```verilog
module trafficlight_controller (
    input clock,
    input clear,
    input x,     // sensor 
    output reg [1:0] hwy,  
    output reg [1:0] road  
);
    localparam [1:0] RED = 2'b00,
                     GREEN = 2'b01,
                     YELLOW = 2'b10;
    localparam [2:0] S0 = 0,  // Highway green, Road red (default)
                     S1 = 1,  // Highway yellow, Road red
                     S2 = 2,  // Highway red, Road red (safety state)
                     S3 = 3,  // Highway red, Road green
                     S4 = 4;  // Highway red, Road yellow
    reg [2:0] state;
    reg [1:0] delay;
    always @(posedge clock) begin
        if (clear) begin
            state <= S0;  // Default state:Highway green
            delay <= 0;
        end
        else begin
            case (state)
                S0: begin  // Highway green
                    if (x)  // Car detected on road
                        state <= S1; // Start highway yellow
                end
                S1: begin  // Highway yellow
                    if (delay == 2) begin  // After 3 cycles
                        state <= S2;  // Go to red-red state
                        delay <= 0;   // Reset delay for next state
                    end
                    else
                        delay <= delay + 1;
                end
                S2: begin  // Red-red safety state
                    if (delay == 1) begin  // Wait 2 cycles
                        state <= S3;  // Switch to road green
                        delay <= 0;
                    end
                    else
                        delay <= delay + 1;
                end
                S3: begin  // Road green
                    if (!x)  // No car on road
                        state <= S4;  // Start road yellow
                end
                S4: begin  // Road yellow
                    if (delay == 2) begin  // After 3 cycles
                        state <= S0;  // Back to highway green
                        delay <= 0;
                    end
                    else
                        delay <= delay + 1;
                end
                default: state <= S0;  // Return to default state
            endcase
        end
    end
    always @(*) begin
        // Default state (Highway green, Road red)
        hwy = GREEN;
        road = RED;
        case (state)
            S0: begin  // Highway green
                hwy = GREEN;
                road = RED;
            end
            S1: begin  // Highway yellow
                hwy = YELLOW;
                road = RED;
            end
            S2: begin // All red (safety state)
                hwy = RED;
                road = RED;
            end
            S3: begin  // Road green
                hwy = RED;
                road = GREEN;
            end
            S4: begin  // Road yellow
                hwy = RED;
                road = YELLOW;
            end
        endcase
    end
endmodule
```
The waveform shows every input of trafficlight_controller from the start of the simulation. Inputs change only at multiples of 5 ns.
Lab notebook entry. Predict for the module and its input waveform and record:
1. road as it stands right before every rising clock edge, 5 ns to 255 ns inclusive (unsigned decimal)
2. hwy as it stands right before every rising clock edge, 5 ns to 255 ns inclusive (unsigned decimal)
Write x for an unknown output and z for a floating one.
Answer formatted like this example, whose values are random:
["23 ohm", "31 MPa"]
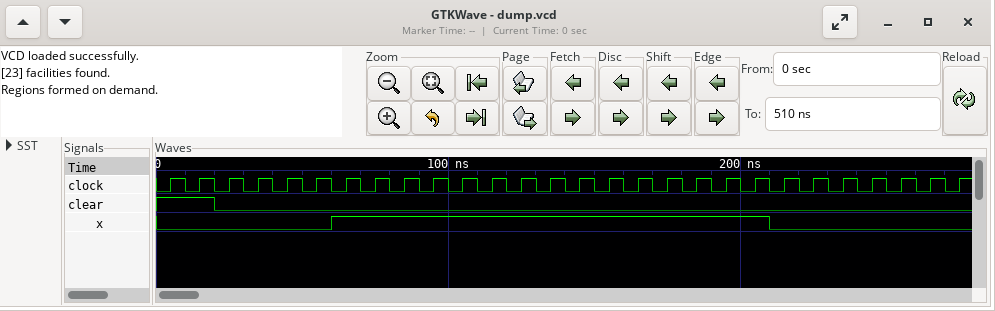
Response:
["x, 0, 0, 0, 0, 0, 0, 0, 0, 0, 0, 0, 1, 1, 1, 1, 1, 1, 1, 1, 1, 1, 2, 2, 2, 0", "x, 1, 1, 1, 1, 1, 1, 2, 2, 2, 0, 0, 0, 0, 0, 0, 0, 0, 0, 0, 0, 0, 0, 0, 0, 1"]
